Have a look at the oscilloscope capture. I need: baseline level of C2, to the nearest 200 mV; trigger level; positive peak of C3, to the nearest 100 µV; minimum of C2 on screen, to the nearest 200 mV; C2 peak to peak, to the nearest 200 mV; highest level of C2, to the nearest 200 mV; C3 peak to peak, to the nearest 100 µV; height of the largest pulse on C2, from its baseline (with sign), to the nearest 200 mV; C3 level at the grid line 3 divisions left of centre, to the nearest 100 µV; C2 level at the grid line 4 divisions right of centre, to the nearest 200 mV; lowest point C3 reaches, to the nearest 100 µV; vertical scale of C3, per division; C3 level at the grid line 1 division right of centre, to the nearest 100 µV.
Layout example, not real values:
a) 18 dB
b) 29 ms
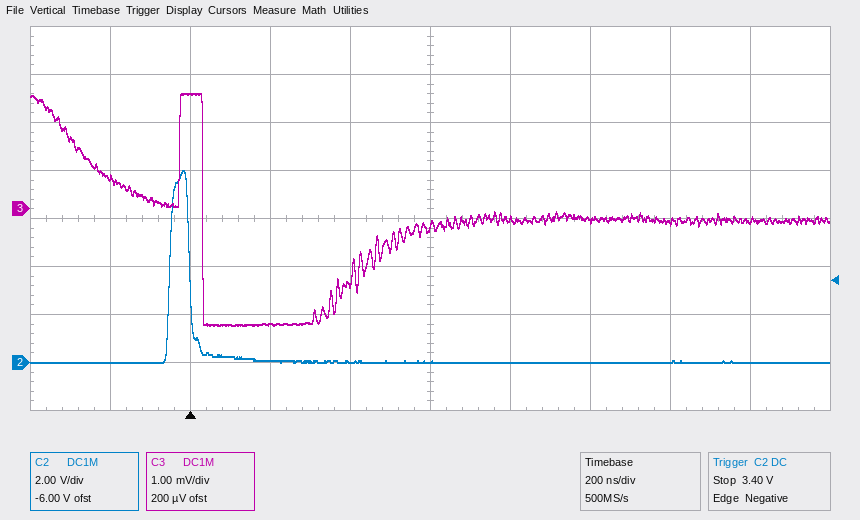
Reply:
a) 0.0 V
b) 3.40 V
c) 2.4 mV
d) 0.0 V
e) 8.0 V
f) 8.0 V
g) 4.8 mV
h) +8.0 V
i) 2.4 mV
j) 0.0 V
k) -2.4 mV
l) 1 mV
m) -200 µV
